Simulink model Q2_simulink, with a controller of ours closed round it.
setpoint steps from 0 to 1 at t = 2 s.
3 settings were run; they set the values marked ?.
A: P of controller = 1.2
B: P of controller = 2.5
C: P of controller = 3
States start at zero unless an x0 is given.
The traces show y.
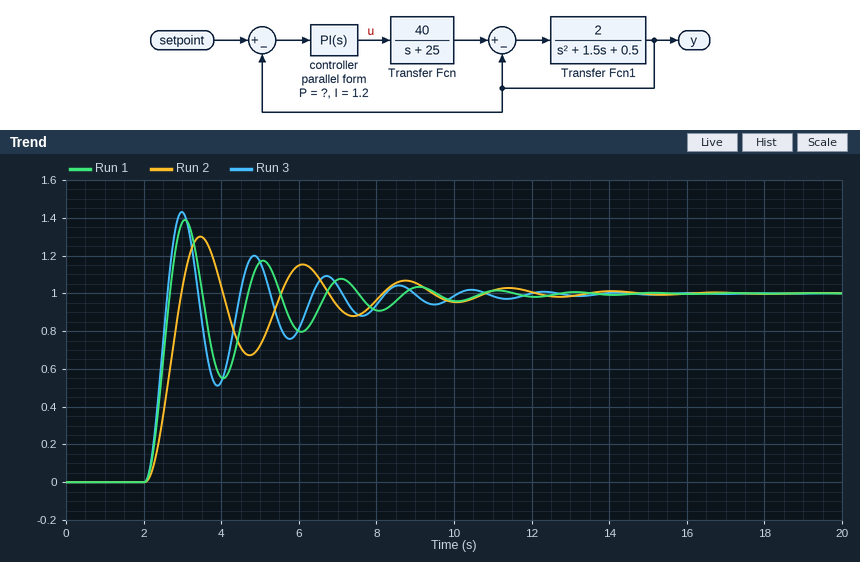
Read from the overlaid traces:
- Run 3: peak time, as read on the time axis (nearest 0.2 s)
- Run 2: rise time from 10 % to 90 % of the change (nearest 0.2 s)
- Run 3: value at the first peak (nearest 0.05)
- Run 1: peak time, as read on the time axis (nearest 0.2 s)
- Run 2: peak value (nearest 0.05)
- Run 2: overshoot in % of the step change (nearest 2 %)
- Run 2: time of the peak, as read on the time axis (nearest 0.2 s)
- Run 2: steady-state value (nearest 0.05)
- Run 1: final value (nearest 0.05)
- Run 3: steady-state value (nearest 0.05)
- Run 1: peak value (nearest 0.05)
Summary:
3.0 s
0.6 s
1.45
3.0 s
1.30
30 %
3.4 s
1.00
1.00
1.00
1.40
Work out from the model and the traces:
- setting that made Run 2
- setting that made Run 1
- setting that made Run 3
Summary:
A
B
C
